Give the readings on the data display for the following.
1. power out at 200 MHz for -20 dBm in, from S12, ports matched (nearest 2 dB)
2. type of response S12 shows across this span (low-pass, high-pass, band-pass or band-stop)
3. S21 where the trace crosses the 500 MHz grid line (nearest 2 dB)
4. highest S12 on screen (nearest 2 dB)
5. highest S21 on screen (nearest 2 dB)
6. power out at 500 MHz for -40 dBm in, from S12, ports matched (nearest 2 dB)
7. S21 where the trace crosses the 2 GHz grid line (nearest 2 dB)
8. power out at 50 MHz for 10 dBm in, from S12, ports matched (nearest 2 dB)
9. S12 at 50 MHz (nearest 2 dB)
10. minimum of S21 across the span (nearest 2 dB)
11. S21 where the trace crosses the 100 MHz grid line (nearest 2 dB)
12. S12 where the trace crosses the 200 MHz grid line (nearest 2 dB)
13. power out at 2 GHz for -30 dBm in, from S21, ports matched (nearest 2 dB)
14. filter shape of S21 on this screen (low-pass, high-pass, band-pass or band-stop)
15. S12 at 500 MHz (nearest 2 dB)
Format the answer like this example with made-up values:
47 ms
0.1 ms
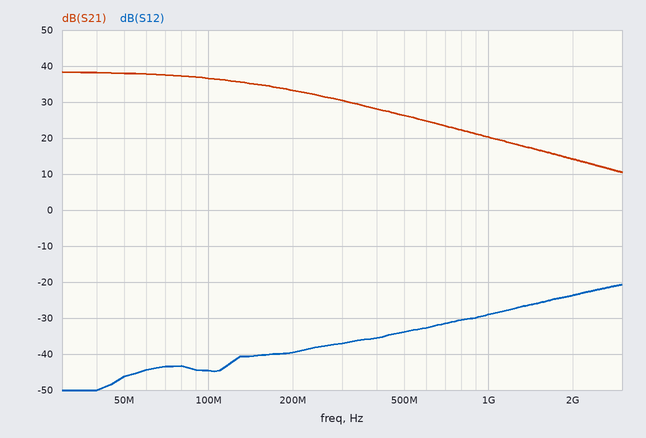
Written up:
-60 dBm
high-pass
26 dB
-20 dB
38 dB
-74 dBm
14 dB
-36 dBm
-46 dB
10 dB
36 dB
-40 dB
-16 dBm
low-pass
-34 dB
